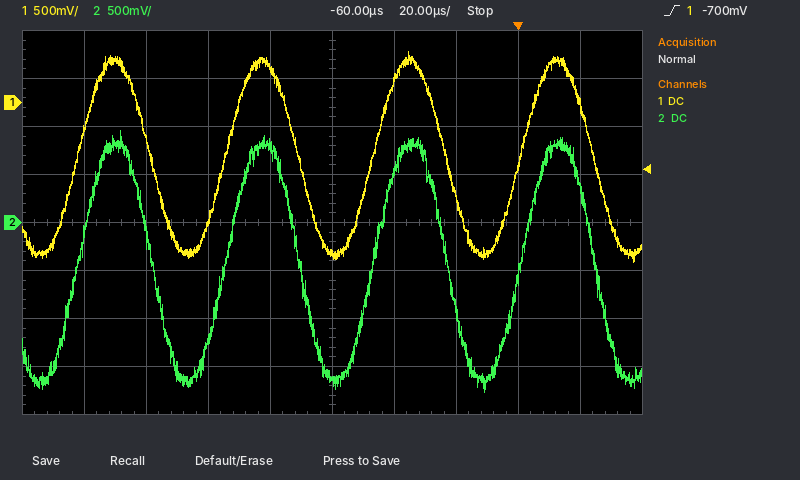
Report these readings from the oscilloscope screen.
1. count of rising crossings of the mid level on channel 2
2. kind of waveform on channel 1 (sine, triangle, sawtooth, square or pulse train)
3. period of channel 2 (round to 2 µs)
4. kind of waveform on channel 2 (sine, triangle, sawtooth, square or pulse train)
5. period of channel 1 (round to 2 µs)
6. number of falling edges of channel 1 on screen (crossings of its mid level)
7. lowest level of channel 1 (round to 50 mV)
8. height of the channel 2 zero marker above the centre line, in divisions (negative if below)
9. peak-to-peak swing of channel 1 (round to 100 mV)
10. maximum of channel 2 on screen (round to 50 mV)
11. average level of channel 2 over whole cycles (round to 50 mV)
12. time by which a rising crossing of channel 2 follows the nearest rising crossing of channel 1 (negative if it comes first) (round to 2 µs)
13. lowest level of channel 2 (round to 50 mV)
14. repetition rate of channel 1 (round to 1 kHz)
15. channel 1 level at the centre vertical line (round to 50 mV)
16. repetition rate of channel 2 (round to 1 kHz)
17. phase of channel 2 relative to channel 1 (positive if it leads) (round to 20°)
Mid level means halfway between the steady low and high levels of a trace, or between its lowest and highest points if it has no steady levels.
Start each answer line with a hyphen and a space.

- 4
- sine
- 48 µs
- sine
- 48 µs
- 4
- -1.65 V
- 0.0 div
- 2.20 V
- 950 mV
- -400 mV
- 0 µs
- -1.75 V
- 21 kHz
- -1.60 V
- 21 kHz
- 0°
